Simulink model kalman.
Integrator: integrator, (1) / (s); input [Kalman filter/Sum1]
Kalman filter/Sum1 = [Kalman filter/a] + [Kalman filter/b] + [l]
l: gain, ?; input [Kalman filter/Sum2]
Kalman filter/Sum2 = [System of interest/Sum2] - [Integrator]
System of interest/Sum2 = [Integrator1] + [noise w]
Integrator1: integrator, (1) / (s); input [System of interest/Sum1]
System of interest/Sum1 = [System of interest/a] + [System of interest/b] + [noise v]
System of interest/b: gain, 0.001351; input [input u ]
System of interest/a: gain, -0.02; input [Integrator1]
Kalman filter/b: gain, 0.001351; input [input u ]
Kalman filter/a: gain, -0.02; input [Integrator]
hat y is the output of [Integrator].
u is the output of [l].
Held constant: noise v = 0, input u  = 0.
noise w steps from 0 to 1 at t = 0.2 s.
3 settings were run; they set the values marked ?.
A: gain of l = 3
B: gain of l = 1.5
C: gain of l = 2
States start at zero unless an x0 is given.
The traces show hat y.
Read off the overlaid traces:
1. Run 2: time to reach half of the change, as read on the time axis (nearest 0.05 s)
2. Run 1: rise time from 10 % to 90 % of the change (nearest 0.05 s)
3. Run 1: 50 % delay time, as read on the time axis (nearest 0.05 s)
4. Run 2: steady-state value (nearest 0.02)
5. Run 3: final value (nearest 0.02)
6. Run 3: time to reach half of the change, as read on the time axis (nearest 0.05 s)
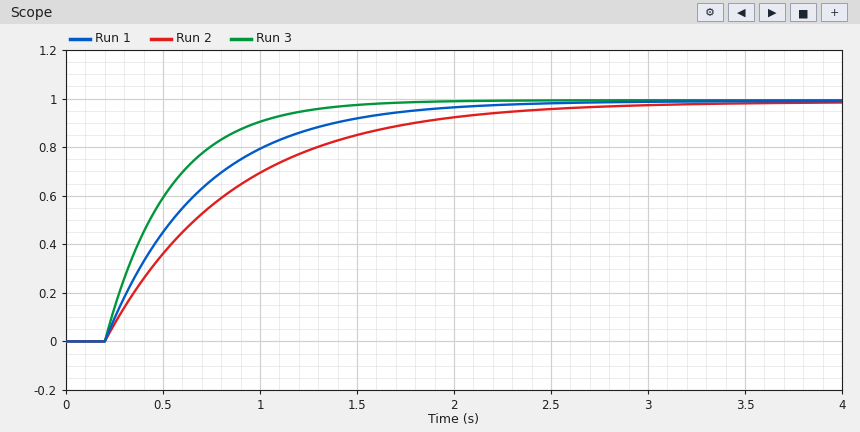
0.65 s
1.10 s
0.55 s
0.98
1.00
0.45 s
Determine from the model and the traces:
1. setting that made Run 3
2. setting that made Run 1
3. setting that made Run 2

A
C
B
